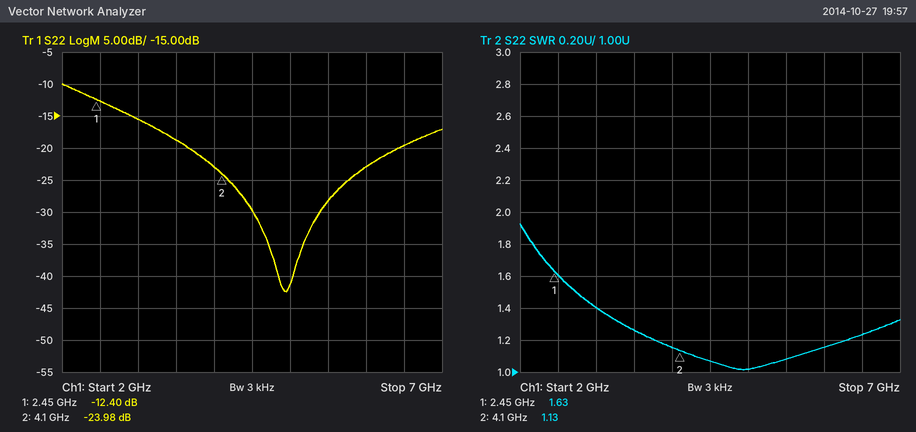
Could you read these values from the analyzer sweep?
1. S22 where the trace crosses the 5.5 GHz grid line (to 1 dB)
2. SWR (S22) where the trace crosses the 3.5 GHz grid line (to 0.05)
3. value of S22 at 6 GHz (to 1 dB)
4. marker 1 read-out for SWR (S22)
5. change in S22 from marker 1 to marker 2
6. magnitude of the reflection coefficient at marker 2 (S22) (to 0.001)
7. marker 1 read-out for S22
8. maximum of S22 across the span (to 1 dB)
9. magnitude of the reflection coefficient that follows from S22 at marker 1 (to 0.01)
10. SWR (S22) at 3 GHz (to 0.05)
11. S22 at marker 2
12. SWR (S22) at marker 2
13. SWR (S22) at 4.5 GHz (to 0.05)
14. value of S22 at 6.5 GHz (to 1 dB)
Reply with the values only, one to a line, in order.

-28 dB
1.25
-23 dB
1.63
-11.58 dB
0.063
-12.40 dB
-10 dB
0.24
1.40
-23.98 dB
1.13
1.05
-20 dB
